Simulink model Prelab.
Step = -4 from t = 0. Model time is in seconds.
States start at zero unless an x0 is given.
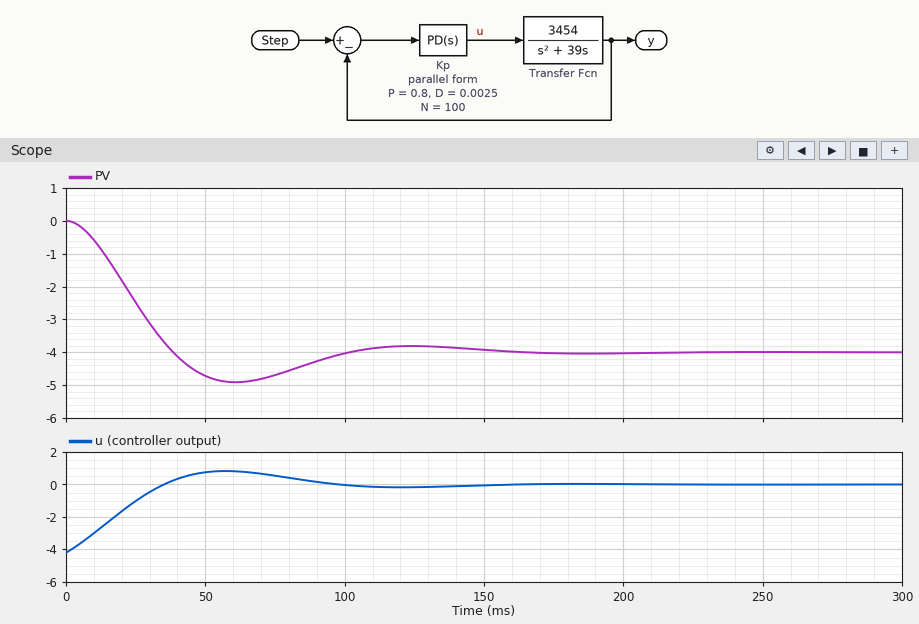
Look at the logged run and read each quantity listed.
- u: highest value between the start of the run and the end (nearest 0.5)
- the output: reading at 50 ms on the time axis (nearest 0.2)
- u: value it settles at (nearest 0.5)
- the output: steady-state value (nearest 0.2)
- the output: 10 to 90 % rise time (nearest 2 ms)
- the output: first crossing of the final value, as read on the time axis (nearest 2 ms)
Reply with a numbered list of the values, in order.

1. 1.0
2. -4.8
3. 0.0
4. -4.0
5. 26 ms
6. 38 ms
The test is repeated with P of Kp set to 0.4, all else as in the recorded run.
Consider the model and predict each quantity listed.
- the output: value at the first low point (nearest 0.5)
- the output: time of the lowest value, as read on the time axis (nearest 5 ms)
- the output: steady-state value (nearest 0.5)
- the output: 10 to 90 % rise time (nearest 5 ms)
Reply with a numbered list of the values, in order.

1. -4.5
2. 95 ms
3. -4.0
4. 45 ms
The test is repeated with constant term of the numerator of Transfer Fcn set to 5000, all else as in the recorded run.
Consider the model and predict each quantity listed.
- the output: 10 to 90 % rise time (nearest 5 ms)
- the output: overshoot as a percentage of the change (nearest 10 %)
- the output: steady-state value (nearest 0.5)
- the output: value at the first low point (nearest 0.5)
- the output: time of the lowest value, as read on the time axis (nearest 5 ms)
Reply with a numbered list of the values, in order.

1. 20 ms
2. 30 %
3. -4.0
4. -5.0
5. 50 ms
